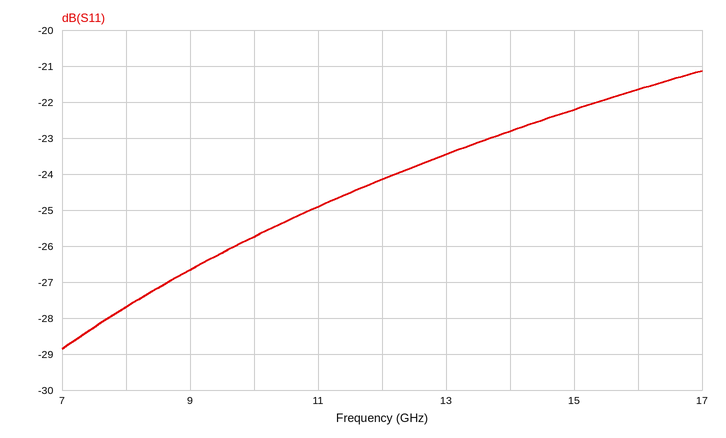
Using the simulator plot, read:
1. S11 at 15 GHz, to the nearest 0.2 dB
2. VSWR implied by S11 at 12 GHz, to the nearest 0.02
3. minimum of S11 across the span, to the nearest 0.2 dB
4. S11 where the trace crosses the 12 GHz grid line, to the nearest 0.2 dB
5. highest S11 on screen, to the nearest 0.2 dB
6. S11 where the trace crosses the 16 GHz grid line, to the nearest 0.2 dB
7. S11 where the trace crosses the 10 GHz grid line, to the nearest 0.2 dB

-22.2 dB
1.14
-28.8 dB
-24.2 dB
-21.2 dB
-21.6 dB
-25.8 dB
